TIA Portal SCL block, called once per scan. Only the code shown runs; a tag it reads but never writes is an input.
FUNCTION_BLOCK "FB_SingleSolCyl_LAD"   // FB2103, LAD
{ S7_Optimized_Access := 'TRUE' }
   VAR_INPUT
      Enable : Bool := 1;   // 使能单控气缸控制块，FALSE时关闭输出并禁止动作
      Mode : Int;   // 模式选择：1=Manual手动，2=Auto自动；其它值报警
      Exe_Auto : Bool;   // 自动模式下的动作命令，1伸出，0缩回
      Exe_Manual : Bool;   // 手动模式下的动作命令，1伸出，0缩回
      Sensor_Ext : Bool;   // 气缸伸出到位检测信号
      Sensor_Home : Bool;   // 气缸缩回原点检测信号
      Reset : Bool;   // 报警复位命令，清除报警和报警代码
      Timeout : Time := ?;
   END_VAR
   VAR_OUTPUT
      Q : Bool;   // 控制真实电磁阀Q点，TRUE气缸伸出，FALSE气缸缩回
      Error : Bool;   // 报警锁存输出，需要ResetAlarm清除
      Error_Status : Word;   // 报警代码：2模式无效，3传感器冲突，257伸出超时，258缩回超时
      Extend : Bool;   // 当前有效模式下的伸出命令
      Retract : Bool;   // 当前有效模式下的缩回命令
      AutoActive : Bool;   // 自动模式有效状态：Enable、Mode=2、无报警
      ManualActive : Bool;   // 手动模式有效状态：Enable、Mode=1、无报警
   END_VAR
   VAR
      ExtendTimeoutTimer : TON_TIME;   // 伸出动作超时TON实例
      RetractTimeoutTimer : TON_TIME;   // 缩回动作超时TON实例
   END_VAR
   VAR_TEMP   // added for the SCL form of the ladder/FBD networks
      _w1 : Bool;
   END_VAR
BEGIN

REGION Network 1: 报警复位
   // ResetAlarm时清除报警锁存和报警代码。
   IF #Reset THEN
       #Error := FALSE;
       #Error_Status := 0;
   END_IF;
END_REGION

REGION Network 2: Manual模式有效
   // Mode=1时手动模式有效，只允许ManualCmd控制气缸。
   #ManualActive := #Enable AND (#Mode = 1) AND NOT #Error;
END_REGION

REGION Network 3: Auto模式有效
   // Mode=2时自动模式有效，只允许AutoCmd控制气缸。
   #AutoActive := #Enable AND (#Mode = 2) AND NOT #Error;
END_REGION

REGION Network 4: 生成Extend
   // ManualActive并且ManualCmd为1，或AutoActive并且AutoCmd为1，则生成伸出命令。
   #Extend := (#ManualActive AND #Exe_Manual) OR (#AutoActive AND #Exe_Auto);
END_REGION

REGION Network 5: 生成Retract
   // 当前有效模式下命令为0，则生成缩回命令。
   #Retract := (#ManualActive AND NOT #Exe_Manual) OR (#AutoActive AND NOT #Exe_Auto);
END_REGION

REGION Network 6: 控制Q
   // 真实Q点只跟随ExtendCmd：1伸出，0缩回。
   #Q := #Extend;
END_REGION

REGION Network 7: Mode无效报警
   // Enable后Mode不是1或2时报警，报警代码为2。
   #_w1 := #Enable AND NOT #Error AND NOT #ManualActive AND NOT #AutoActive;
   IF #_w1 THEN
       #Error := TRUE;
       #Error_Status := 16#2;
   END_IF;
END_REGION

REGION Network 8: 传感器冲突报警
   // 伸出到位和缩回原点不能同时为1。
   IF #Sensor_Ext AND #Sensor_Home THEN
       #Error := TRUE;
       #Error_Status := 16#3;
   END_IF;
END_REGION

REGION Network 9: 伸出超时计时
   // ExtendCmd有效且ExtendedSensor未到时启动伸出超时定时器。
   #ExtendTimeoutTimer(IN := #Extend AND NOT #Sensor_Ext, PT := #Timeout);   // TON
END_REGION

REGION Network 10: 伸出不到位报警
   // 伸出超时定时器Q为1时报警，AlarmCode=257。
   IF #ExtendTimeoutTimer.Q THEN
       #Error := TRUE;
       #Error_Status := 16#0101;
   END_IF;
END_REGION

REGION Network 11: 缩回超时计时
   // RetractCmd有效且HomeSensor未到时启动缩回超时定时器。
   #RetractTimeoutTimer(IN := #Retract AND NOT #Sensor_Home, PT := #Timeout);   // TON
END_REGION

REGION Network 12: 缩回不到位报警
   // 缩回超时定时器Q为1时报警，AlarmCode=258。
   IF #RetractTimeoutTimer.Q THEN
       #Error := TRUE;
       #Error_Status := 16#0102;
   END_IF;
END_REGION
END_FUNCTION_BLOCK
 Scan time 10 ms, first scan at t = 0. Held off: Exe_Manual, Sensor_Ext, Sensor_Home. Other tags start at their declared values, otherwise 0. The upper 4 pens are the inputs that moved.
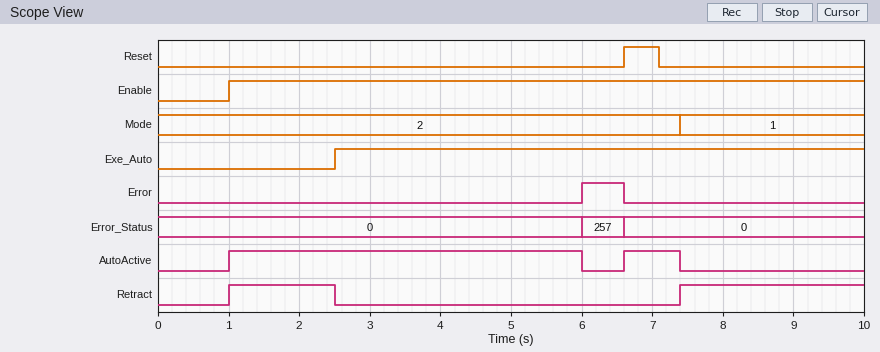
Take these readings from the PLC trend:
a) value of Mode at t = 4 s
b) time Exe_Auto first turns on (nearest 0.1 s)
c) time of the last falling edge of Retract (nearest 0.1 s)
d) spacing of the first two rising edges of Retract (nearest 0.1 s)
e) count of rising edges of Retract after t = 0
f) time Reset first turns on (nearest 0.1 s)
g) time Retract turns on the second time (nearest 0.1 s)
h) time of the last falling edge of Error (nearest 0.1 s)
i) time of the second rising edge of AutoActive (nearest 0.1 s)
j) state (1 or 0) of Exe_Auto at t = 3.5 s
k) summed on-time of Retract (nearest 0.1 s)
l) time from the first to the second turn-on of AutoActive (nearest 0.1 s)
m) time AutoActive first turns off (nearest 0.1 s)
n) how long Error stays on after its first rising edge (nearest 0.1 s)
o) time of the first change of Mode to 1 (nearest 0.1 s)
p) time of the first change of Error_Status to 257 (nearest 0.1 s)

2
2.5 s
2.5 s
6.4 s
2
6.6 s
7.4 s
6.6 s
6.6 s
1
4.1 s
5.6 s
6.0 s
0.6 s
7.4 s
6.0 s
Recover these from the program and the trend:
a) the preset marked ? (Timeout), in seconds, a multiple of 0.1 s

3.5 s
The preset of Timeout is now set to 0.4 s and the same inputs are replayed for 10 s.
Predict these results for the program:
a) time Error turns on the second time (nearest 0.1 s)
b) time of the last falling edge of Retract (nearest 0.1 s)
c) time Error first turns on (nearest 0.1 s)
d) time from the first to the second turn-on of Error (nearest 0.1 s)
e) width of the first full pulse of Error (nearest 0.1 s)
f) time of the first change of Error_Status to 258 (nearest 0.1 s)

7.0 s
1.4 s
1.4 s
5.6 s
5.2 s
1.4 s
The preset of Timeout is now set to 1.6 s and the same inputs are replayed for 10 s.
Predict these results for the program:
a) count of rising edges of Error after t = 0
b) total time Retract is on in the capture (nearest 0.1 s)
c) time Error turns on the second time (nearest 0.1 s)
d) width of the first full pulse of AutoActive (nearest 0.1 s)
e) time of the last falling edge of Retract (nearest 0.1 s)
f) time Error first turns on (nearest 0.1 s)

2
3.1 s
9.0 s
3.1 s
9.0 s
4.1 s
